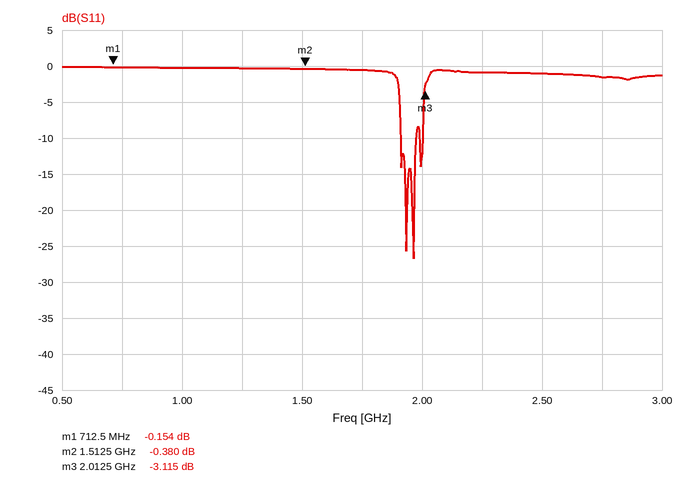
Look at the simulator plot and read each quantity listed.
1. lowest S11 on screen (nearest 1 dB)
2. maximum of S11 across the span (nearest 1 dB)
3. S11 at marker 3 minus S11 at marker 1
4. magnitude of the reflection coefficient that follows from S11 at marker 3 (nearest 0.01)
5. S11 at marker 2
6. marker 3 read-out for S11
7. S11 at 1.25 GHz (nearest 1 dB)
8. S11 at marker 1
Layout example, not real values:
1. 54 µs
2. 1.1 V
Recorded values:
1. -27 dB
2. 0 dB
3. -2.961 dB
4. 0.70
5. -0.380 dB
6. -3.115 dB
7. 0 dB
8. -0.154 dB
